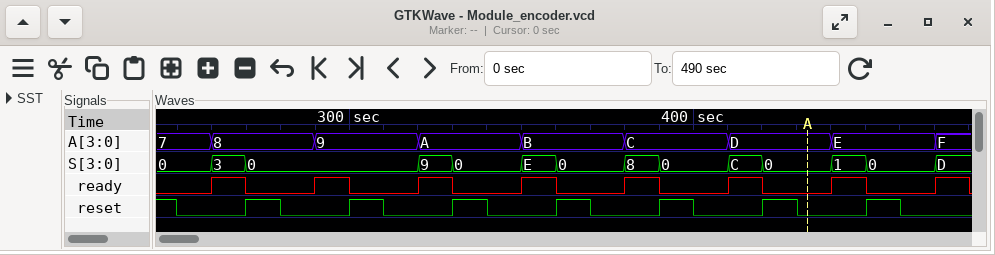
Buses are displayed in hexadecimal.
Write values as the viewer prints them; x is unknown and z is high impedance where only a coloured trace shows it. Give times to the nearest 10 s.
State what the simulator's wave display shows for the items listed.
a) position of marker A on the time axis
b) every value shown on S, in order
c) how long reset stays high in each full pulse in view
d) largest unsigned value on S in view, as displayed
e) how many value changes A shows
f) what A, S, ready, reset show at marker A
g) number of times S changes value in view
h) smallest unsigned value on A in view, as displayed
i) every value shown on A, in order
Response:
430 s
0, 3, 0, 9, 0, E, 0, 8, 0, C, 0, 1, 0, D
10 s, 10 s, 10 s, 10 s, 10 s, 10 s, 10 s
E
8
A=D, S=0, ready=0, reset=0
13
7
7, 8, 9, A, B, C, D, E, F
